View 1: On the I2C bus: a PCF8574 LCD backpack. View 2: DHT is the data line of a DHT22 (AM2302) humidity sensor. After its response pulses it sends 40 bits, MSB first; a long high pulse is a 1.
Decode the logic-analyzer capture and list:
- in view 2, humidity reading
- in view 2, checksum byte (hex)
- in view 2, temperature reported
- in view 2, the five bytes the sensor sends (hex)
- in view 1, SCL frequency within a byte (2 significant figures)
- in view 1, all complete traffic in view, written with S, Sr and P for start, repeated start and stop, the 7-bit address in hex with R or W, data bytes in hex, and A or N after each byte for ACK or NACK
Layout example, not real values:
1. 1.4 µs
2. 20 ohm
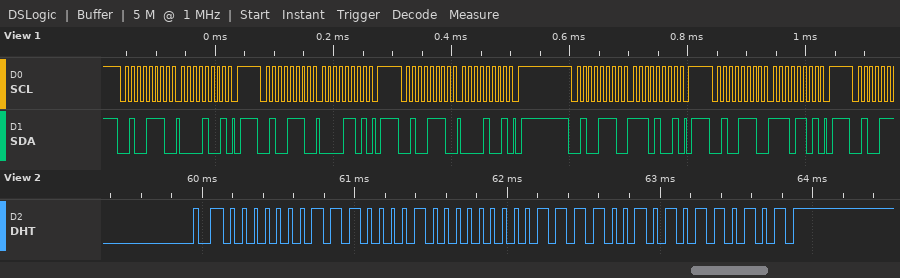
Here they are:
1. 45.0 %
2. 0xB5
3. 24.2 °C
4. 01 C2 00 F2 B5
5. 100 kHz
6. S 27W A 09 A P S 27W A 0D A P S 27W A 09 A P S 27W A E9 A P S 27W A ED A P
